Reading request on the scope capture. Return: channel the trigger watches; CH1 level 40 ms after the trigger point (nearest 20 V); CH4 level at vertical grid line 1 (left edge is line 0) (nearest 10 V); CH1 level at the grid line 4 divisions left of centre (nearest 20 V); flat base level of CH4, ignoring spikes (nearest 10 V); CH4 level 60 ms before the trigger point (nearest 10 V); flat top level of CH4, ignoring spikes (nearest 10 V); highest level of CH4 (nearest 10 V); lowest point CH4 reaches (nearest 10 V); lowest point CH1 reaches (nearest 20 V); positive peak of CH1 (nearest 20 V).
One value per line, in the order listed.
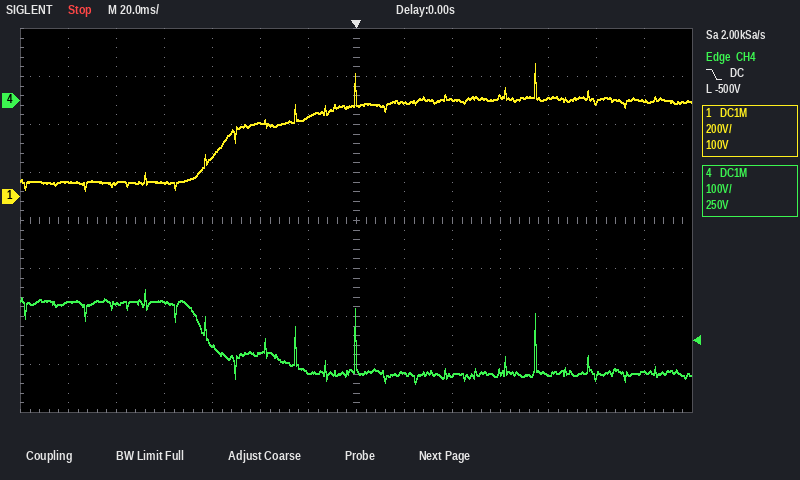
CH4
400 V
-420 V
60 V
-570 V
-510 V
-420 V
-390 V
-590 V
20 V
560 V
